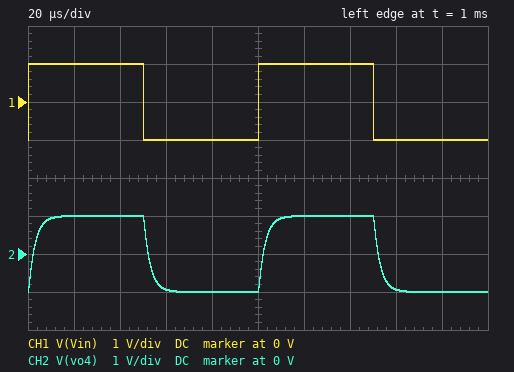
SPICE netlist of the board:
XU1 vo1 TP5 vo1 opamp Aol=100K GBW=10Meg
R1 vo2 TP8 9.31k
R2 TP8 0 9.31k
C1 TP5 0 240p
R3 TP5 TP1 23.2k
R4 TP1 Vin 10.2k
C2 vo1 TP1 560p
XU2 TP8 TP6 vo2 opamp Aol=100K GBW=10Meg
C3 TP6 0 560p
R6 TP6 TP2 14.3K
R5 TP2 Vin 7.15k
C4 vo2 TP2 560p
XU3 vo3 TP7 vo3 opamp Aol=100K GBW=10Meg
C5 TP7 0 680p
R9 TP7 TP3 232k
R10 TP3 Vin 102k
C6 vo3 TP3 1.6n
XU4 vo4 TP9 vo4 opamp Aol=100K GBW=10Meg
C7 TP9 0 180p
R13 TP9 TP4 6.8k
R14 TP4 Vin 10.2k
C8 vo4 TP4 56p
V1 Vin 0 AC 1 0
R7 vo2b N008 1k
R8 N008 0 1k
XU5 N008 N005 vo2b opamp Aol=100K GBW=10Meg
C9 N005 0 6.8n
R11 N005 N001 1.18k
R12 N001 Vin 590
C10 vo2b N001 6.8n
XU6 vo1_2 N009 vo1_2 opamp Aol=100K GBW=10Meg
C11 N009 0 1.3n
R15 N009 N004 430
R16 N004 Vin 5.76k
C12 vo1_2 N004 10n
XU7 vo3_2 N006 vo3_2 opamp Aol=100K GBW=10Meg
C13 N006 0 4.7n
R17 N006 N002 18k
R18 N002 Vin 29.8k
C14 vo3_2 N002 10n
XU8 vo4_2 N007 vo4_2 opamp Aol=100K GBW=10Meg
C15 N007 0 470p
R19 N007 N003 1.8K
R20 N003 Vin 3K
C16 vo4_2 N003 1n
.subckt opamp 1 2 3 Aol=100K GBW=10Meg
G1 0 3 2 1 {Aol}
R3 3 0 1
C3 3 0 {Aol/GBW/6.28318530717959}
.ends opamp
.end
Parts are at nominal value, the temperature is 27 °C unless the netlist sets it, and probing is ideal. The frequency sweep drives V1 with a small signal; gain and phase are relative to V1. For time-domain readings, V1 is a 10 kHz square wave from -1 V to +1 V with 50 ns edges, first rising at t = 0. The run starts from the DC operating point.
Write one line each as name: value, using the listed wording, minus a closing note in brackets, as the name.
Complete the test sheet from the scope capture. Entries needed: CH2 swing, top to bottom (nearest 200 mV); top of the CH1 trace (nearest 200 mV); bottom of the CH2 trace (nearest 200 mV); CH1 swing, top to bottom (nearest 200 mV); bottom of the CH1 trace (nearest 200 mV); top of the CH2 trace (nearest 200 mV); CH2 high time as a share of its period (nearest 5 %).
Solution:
CH2 swing, top to bottom: 2.0 V
top of the CH1 trace: 1.0 V
bottom of the CH2 trace: -1.0 V
CH1 swing, top to bottom: 2.0 V
bottom of the CH1 trace: -1.0 V
top of the CH2 trace: 1.0 V
CH2 high time as a share of its period: 50 %
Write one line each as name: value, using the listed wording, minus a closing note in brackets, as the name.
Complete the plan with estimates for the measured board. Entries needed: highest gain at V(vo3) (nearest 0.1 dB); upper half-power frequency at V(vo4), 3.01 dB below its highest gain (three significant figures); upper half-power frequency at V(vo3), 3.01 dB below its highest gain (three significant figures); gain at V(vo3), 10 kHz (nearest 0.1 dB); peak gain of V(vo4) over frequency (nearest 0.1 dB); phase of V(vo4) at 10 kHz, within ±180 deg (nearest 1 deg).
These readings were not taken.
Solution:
highest gain at V(vo3): 0 dB
upper half-power frequency at V(vo4), 3.01 dB below its highest gain: 56.2 kHz
upper half-power frequency at V(vo3), 3.01 dB below its highest gain: 991 Hz
gain at V(vo3), 10 kHz: -40.1 dB
peak gain of V(vo4) over frequency: 0 dB
phase of V(vo4) at 10 kHz, within ±180 deg: -11 deg
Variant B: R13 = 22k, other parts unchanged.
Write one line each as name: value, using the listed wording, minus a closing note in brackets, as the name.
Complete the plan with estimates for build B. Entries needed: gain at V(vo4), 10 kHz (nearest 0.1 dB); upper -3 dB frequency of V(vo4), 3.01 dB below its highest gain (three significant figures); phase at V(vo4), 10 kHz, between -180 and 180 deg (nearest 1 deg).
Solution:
gain at V(vo4), 10 kHz: -0.5 dB
upper -3 dB frequency of V(vo4), 3.01 dB below its highest gain: 29.4 kHz
phase at V(vo4), 10 kHz, between -180 and 180 deg: -20 deg
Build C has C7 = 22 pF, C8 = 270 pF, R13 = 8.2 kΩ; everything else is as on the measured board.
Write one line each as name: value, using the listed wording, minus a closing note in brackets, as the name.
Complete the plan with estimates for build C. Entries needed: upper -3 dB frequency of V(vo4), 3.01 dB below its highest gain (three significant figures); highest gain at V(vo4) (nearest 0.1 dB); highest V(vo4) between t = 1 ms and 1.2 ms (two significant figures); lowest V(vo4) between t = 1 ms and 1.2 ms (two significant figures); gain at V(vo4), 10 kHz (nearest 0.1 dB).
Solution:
upper -3 dB frequency of V(vo4), 3.01 dB below its highest gain: 254 kHz
highest gain at V(vo4): 5.5 dB
highest V(vo4) between t = 1 ms and 1.2 ms: 1.8 V
lowest V(vo4) between t = 1 ms and 1.2 ms: -1.8 V
gain at V(vo4), 10 kHz: 0 dB
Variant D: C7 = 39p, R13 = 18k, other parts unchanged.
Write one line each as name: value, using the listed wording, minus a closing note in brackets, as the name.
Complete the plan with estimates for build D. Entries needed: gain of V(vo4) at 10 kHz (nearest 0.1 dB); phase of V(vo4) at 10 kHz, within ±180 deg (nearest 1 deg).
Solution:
gain of V(vo4) at 10 kHz: 0 dB
phase of V(vo4) at 10 kHz, within ±180 deg: -4 deg
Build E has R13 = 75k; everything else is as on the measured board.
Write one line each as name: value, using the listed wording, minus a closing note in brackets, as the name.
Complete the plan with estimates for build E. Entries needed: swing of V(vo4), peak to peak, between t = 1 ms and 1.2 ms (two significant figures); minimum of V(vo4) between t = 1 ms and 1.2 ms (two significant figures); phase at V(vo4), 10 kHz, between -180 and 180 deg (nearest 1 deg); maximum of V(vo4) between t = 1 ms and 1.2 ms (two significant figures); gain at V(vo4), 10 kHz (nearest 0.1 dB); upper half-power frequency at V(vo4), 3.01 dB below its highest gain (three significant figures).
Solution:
swing of V(vo4), peak to peak, between t = 1 ms and 1.2 ms: 1.9 V
minimum of V(vo4) between t = 1 ms and 1.2 ms: -930 mV
phase at V(vo4), 10 kHz, between -180 and 180 deg: -45 deg
maximum of V(vo4) between t = 1 ms and 1.2 ms: 930 mV
gain at V(vo4), 10 kHz: -2.7 dB
upper half-power frequency at V(vo4), 3.01 dB below its highest gain: 10.7 kHz
